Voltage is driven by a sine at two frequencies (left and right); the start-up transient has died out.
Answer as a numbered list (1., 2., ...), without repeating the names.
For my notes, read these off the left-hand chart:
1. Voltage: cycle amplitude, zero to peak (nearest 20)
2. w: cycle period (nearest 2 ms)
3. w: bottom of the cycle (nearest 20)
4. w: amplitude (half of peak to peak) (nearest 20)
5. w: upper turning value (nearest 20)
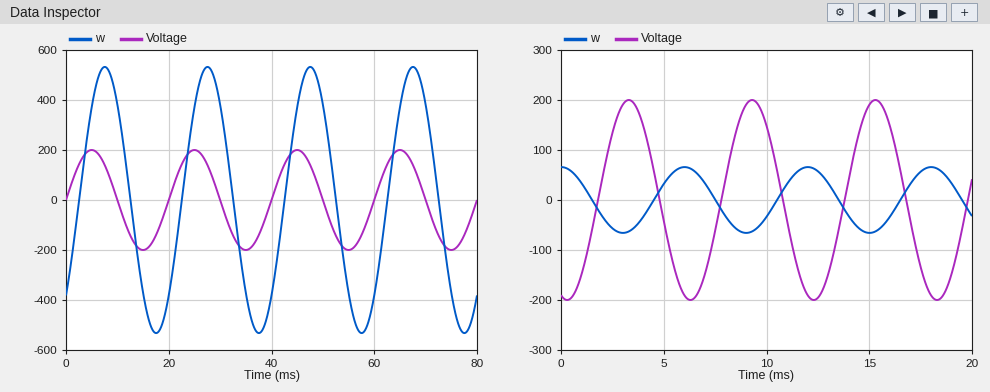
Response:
1. 200
2. 20 ms
3. -540
4. 540
5. 540
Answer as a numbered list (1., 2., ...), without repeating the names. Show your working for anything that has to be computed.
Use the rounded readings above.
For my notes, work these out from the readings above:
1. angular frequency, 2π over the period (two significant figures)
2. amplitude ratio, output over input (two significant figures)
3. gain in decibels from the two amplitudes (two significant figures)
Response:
1. 2π / 20 = 0.31 rad/ms
2. 540 / 200 = 2.7
3. 20 log10(540 / 200) = 8.6 dB
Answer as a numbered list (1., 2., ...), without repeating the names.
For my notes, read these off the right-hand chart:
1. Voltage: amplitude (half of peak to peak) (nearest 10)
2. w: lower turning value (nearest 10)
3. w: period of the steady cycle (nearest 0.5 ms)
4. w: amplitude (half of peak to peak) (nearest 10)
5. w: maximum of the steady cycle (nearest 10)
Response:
1. 200
2. -70
3. 6.0 ms
4. 70
5. 70
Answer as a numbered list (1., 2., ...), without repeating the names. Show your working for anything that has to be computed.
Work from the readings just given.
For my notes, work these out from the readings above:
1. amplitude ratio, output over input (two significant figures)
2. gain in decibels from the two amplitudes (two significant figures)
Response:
1. 70 / 200 = 0.35
2. 20 log10(70 / 200) = -9.1 dB
